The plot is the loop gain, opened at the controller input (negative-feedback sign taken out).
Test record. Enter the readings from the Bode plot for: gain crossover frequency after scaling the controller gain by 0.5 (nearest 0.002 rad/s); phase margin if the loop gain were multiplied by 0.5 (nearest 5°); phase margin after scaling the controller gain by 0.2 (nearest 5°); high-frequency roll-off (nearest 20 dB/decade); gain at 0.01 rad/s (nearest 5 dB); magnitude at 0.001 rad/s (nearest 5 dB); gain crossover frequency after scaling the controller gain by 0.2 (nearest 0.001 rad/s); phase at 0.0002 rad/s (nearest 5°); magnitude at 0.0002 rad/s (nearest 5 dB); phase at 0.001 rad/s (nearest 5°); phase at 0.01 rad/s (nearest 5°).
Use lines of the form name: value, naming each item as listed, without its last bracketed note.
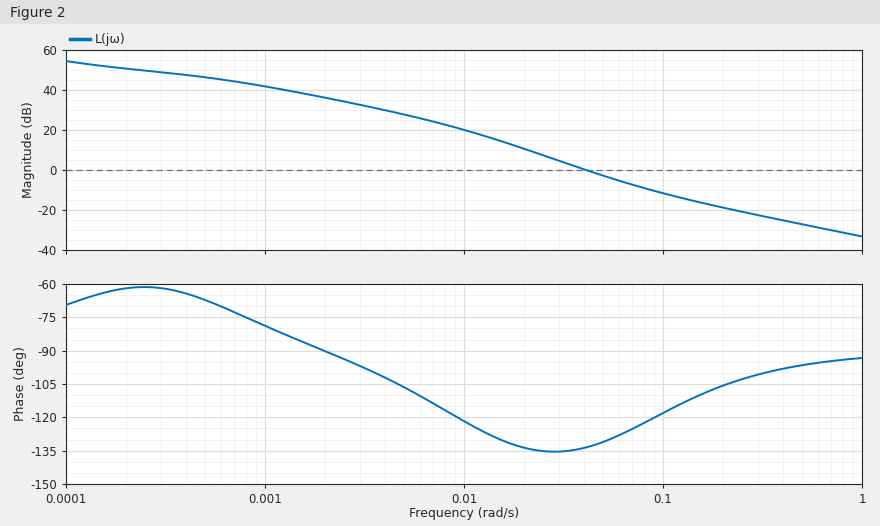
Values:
gain crossover frequency after scaling the controller gain by 0.5: 0.028 rad/s
phase margin if the loop gain were multiplied by 0.5: 45°
phase margin after scaling the controller gain by 0.2: 50°
high-frequency roll-off: -20 dB/decade
gain at 0.01 rad/s: 20 dB
magnitude at 0.001 rad/s: 40 dB
gain crossover frequency after scaling the controller gain by 0.2: 0.016 rad/s
phase at 0.0002 rad/s: -60°
magnitude at 0.0002 rad/s: 50 dB
phase at 0.001 rad/s: -80°
phase at 0.01 rad/s: -120°
